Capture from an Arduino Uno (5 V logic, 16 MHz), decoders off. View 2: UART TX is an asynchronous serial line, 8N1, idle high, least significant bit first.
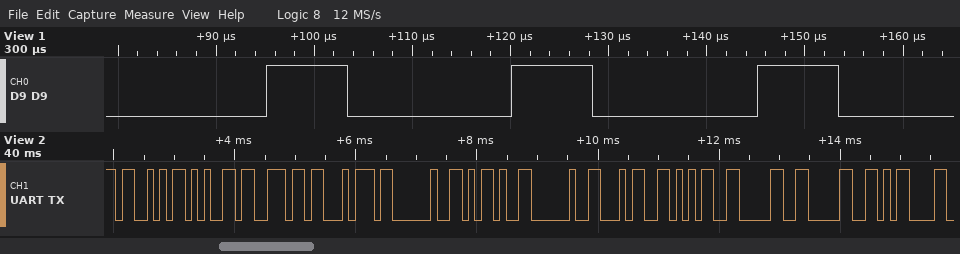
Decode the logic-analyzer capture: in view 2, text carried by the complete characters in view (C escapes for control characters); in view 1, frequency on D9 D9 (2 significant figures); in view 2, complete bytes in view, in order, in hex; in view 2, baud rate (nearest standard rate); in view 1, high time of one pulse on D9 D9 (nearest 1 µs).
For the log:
"Sent - 4500\r"
40 kHz
0x53 0x65 0x6E 0x74 0x20 0x2D 0x20 0x34 0x35 0x30 0x30 0x0D
9600 baud
8 µs
